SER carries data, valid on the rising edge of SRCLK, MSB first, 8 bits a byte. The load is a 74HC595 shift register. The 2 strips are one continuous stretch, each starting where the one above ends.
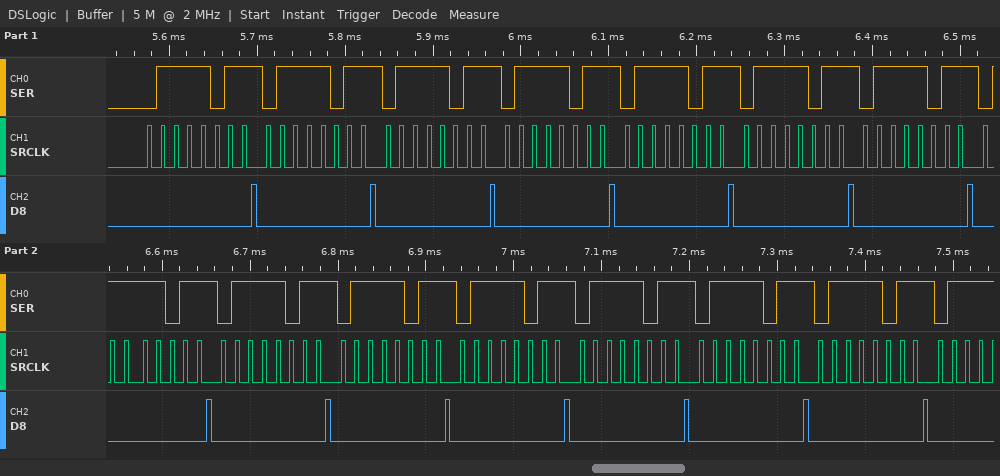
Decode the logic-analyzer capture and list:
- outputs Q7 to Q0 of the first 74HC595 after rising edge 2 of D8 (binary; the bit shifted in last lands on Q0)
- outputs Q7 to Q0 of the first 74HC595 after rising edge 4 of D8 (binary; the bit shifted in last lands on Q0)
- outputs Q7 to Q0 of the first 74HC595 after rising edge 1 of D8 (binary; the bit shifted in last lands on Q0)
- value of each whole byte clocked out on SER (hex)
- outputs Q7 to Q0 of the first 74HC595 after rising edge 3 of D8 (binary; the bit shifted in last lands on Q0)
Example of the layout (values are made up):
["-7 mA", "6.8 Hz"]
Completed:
["01111011", "01111011", "01111011", "7B 7B 7B 7B 7B 7B 7B 7B 7B 7B 7B 7B 7B 7B", "01111011"]
